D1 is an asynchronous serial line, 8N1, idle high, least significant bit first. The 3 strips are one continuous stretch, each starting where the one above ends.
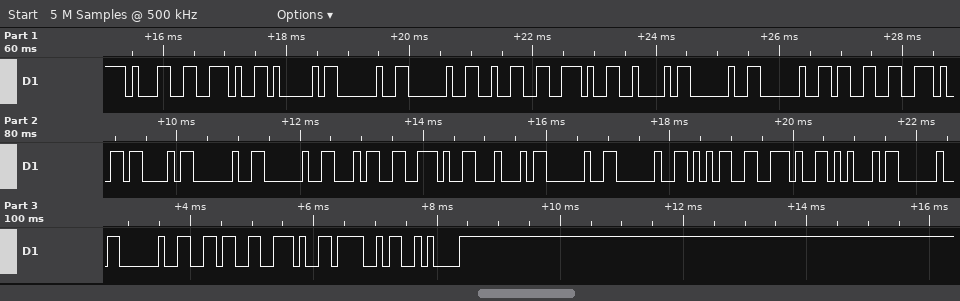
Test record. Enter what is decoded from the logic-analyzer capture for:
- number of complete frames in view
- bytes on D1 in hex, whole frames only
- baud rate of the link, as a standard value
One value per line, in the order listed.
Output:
29
31 2E 41 20 20 32 2E 42 20 20 33 2E 43 20 20 34 2E 44 20 20 35 2E 45 20 20 36 2E 4F 0A
9600 baud
